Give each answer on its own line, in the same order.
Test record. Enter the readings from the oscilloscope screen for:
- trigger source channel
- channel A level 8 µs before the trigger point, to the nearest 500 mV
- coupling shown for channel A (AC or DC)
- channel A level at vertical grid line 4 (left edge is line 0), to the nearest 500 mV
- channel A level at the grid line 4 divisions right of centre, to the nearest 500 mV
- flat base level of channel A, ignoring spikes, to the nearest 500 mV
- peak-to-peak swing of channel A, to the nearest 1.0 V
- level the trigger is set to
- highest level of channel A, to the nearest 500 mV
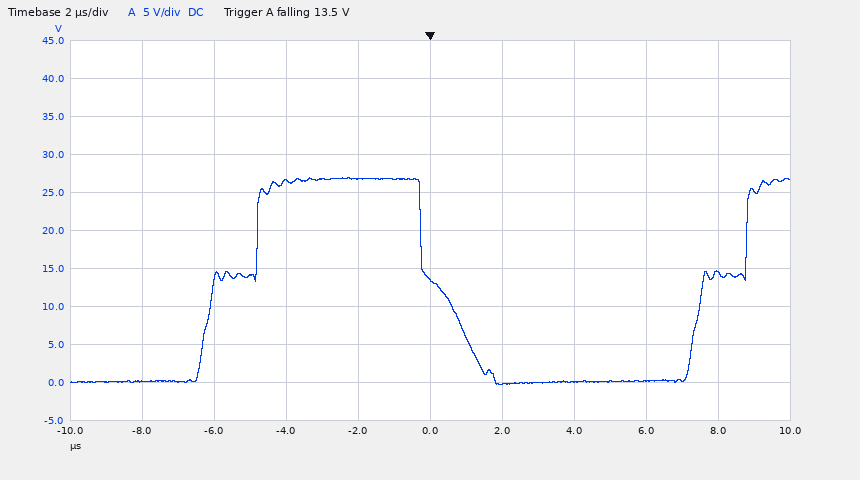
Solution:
channel A
0.0 V
DC
27.0 V
14.5 V
0.0 V
27.0 V
13.5 V
27.0 V
